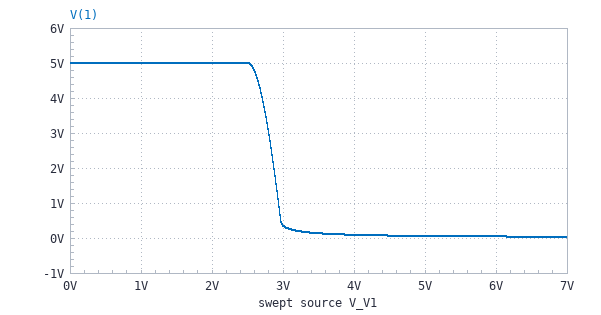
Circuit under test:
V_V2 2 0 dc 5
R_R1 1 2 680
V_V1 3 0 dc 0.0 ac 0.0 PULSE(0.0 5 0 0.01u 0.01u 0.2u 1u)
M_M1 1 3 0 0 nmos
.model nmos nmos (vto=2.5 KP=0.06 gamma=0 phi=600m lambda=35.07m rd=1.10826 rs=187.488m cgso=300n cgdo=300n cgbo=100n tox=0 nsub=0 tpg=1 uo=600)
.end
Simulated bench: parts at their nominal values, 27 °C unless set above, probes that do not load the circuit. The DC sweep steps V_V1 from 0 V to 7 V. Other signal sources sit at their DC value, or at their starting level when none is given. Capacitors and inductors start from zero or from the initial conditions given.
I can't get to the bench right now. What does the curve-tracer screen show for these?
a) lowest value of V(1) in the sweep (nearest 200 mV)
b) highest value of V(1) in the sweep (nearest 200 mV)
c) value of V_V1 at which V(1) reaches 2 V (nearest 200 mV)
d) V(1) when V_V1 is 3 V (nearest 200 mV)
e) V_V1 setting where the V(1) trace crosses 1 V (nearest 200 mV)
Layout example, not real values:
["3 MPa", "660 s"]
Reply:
["0 V", "5.0 V", "2.8 V", "400 mV", "3.0 V"]
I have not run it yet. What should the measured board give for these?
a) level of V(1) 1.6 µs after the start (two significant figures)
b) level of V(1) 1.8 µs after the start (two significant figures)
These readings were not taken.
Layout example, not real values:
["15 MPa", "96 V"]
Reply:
["5.0 V", "5.0 V"]
